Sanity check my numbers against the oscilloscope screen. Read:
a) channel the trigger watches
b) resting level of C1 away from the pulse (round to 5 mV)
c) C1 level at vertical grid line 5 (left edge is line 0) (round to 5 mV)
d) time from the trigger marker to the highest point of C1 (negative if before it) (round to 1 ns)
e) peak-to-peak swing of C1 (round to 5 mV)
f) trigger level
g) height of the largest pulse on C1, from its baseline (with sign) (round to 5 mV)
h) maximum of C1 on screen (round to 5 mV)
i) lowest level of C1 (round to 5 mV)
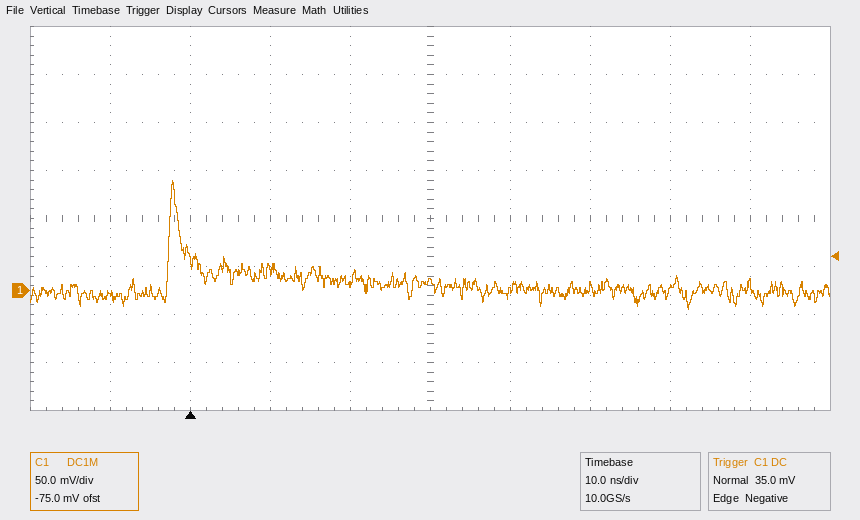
C1
0 mV
10 mV
-2 ns
135 mV
35.0 mV
+115 mV
115 mV
-20 mV
